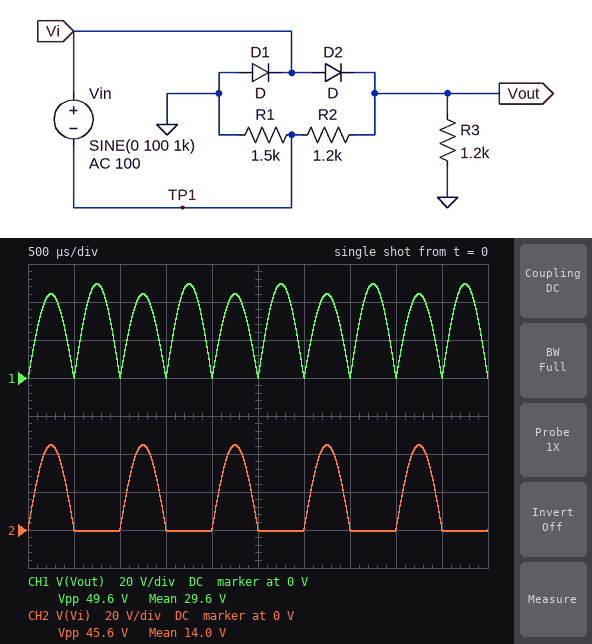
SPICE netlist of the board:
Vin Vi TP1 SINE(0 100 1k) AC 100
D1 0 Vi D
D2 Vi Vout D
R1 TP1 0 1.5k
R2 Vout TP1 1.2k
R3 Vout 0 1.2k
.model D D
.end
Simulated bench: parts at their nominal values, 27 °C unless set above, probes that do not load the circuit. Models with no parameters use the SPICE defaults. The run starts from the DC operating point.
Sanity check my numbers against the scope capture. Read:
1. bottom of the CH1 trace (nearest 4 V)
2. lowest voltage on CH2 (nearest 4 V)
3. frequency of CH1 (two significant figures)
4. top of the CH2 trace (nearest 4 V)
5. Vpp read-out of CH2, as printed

0 V
0 V
2.0 kHz
44 V
45.6 V
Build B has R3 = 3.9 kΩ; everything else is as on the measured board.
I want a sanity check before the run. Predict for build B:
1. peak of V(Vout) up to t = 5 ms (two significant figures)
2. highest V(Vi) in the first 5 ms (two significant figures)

76 V
72 V
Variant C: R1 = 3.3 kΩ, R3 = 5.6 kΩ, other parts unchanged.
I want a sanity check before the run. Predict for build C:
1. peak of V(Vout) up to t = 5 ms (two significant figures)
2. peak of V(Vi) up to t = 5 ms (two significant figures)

82 V
63 V
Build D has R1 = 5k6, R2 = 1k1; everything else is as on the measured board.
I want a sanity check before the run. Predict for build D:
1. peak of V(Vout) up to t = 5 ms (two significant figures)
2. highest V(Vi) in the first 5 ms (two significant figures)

52 V
18 V
